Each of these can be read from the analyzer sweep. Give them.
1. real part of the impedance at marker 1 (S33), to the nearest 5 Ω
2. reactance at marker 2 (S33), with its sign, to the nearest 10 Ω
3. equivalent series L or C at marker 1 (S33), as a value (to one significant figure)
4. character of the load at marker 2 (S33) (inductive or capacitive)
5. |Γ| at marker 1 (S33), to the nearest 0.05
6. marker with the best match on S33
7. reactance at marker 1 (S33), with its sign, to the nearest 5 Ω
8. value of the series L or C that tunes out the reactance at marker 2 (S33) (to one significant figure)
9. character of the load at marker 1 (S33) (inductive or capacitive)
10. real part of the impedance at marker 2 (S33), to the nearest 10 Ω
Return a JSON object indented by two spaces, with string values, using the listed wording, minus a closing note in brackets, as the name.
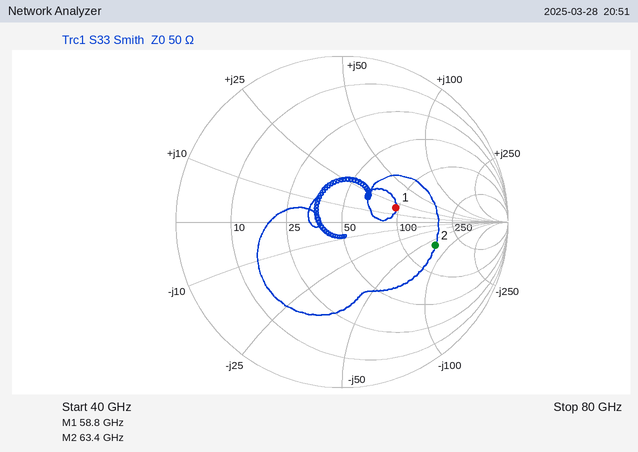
{
  "real part of the impedance at marker 1 (S33), to the nearest 5 Ω": "95 Ω",
  "reactance at marker 2 (S33), with its sign, to the nearest 10 Ω": "-70 Ω",
  "equivalent series L or C at marker 1 (S33), as a value": "50 pH",
  "character of the load at marker 2 (S33)": "capacitive",
  "|Γ| at marker 1 (S33), to the nearest 0.05": "0.35",
  "marker with the best match on S33": "marker 1",
  "reactance at marker 1 (S33), with its sign, to the nearest 5 Ω": "+20 Ω",
  "value of the series L or C that tunes out the reactance at marker 2 (S33)": "200 pH",
  "character of the load at marker 1 (S33)": "inductive",
  "real part of the impedance at marker 2 (S33), to the nearest 10 Ω": "160 Ω"
}
